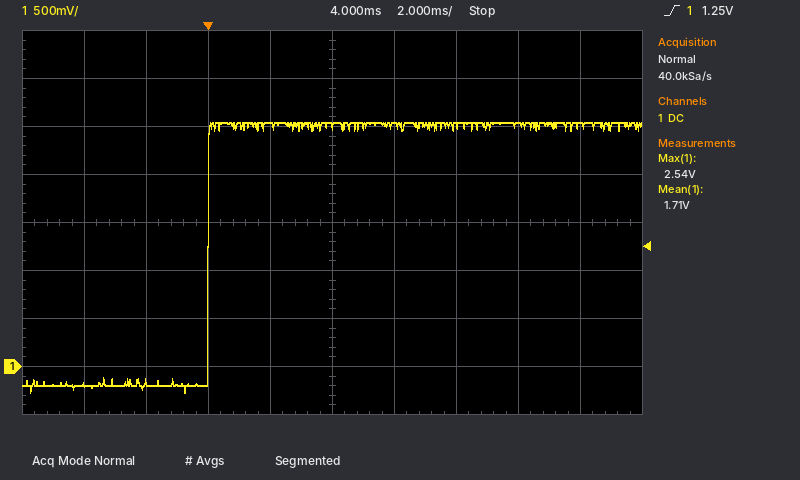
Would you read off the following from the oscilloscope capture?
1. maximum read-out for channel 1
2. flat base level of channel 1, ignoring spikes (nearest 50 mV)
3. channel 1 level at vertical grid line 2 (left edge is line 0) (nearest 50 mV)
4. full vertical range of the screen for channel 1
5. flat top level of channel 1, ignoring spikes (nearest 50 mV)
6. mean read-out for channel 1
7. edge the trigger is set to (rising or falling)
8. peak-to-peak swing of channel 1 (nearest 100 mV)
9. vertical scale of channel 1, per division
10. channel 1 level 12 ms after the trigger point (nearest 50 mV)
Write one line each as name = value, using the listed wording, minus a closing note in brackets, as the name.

maximum read-out for channel 1 = 2.54 V
flat base level of channel 1, ignoring spikes = -200 mV
channel 1 level at vertical grid line 2 (left edge is line 0) = -150 mV
full vertical range of the screen for channel 1 = 4 V
flat top level of channel 1, ignoring spikes = 2.55 V
mean read-out for channel 1 = 1.71 V
edge the trigger is set to = rising
peak-to-peak swing of channel 1 = 2.80 V
vertical scale of channel 1, per division = 500 mV
channel 1 level 12 ms after the trigger point = 2.50 V
